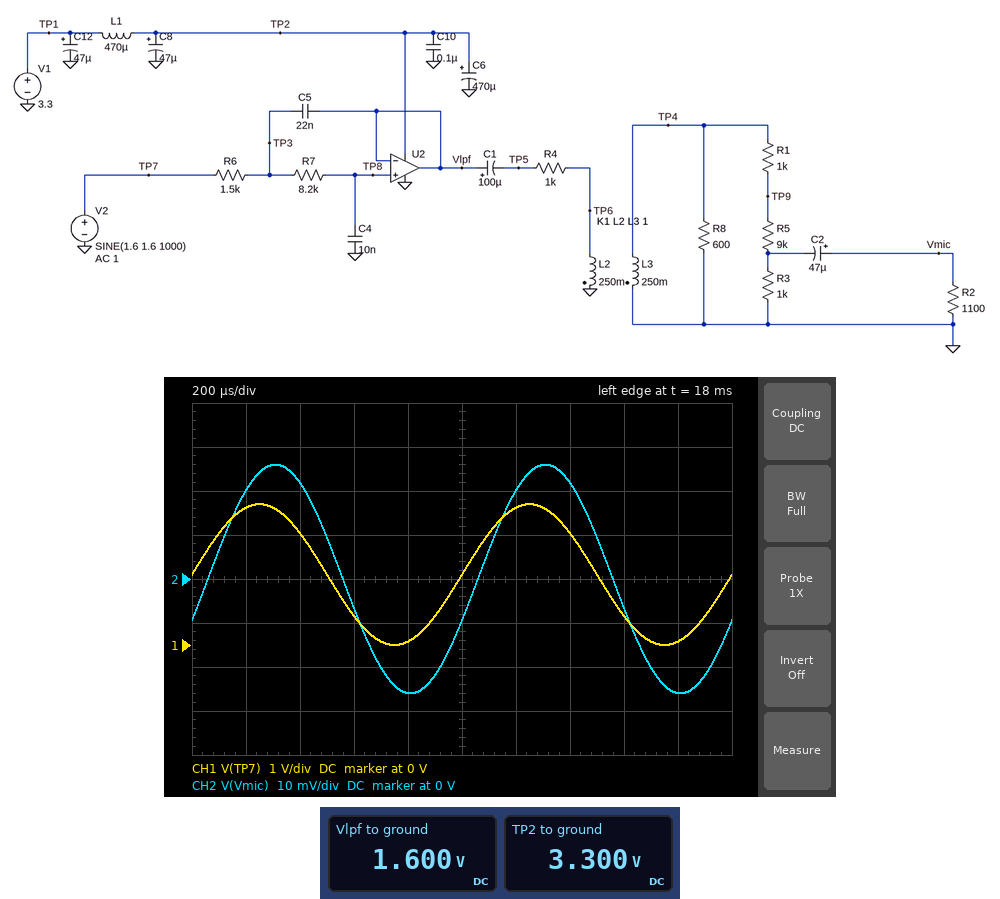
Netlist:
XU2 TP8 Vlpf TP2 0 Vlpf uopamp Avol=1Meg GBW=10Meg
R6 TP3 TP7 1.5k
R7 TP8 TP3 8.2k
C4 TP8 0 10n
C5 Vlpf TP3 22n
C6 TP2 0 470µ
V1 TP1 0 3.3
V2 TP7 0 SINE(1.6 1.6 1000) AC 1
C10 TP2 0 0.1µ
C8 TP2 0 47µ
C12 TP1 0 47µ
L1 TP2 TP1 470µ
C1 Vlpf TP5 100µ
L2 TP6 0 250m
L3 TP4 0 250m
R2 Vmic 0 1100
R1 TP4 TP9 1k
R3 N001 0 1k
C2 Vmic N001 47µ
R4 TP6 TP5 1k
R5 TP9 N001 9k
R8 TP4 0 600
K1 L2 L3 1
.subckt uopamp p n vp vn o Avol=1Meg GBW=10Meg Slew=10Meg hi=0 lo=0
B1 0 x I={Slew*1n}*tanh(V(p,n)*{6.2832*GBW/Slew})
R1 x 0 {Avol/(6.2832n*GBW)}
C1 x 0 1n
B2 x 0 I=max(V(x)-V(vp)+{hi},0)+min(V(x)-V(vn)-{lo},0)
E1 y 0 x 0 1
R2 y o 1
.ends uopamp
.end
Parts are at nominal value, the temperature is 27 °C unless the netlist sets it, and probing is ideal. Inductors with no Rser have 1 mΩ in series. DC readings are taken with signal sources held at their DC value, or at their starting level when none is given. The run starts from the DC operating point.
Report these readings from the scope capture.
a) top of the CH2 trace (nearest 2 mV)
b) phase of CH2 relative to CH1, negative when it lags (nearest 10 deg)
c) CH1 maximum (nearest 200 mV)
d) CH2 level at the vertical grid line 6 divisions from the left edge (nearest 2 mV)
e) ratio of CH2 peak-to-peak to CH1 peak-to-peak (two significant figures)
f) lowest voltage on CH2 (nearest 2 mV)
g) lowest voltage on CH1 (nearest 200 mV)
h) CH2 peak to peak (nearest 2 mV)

26 mV
-20 deg
3.2 V
20 mV
0.016
-26 mV
0 V
52 mV
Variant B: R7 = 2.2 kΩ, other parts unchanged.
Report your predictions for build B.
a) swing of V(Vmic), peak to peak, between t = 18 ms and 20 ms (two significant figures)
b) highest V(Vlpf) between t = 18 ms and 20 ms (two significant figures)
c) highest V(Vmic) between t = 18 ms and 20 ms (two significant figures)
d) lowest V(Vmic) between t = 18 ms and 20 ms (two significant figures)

56 mV
3.2 V
28 mV
-28 mV
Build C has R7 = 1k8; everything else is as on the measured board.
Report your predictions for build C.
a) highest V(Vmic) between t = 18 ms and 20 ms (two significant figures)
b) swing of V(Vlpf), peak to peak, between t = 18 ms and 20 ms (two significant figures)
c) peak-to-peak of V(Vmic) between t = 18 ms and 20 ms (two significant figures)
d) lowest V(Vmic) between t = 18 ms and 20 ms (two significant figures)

28 mV
3.2 V
56 mV
-28 mV
